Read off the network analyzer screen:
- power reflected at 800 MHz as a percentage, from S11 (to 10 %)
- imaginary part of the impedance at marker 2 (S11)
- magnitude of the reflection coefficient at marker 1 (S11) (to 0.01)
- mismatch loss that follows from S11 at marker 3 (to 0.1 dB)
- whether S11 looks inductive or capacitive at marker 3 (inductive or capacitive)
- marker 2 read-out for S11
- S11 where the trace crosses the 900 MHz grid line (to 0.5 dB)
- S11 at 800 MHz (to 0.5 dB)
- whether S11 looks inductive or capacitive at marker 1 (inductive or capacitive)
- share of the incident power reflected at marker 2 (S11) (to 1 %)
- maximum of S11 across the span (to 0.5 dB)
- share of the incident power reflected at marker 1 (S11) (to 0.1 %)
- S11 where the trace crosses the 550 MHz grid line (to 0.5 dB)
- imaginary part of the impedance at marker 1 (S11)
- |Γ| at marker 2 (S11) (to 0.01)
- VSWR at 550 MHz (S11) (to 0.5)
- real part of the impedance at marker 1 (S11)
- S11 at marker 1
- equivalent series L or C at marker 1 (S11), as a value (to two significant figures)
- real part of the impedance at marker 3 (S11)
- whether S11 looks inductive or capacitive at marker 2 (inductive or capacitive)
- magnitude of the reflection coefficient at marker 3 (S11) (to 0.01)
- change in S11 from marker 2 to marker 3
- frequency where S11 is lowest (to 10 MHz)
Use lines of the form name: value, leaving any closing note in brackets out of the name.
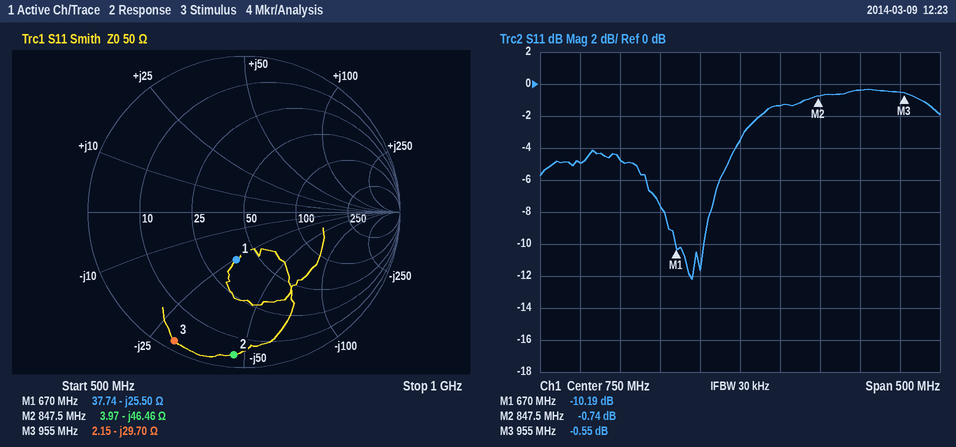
power reflected at 800 MHz as a percentage, from S11: 70 %
imaginary part of the impedance at marker 2: -46.46 Ω
magnitude of the reflection coefficient at marker 1 (S11): 0.31
mismatch loss that follows from S11 at marker 3: 9.2 dB
whether S11 looks inductive or capacitive at marker 3: capacitive
marker 2 read-out for S11: -0.74 dB
S11 where the trace crosses the 900 MHz grid line: -0.5 dB
S11 at 800 MHz: -1.5 dB
whether S11 looks inductive or capacitive at marker 1: capacitive
share of the incident power reflected at marker 2 (S11): 84 %
maximum of S11 across the span: -0.5 dB
share of the incident power reflected at marker 1 (S11): 9.6 %
S11 where the trace crosses the 550 MHz grid line: -5.0 dB
imaginary part of the impedance at marker 1: -25.50 Ω
|Γ| at marker 2 (S11): 0.92
VSWR at 550 MHz (S11): 3.5
real part of the impedance at marker 1: 37.74 Ω
S11 at marker 1: -10.19 dB
equivalent series L or C at marker 1 (S11), as a value: 9.3 pF
real part of the impedance at marker 3: 2.15 Ω
whether S11 looks inductive or capacitive at marker 2: capacitive
magnitude of the reflection coefficient at marker 3 (S11): 0.94
change in S11 from marker 2 to marker 3: 0.19 dB
frequency where S11 is lowest: 690 MHz
